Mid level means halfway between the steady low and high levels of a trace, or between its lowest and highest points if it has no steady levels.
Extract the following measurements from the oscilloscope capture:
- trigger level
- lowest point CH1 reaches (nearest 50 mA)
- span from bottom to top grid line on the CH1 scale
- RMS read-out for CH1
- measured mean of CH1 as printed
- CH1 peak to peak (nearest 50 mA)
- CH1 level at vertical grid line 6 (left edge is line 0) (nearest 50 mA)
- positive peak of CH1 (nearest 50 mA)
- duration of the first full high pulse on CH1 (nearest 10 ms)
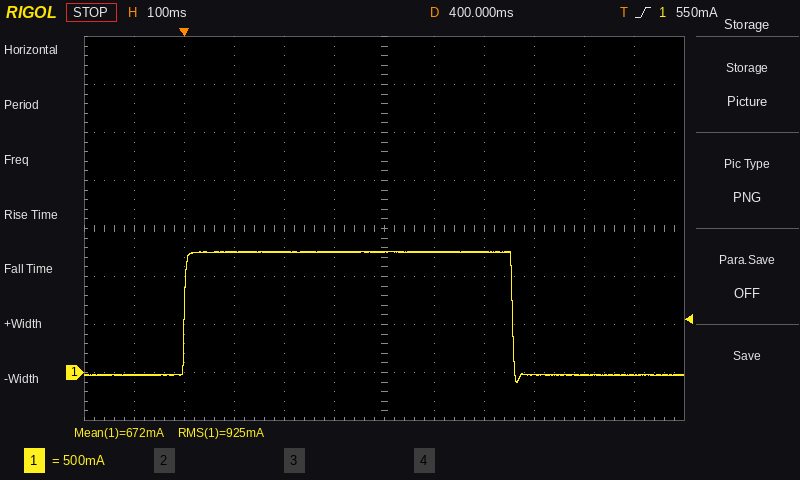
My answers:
550 mA
-100 mA
4 A
925 mA
672 mA
1.35 A
1.25 A
1.25 A
660 ms
